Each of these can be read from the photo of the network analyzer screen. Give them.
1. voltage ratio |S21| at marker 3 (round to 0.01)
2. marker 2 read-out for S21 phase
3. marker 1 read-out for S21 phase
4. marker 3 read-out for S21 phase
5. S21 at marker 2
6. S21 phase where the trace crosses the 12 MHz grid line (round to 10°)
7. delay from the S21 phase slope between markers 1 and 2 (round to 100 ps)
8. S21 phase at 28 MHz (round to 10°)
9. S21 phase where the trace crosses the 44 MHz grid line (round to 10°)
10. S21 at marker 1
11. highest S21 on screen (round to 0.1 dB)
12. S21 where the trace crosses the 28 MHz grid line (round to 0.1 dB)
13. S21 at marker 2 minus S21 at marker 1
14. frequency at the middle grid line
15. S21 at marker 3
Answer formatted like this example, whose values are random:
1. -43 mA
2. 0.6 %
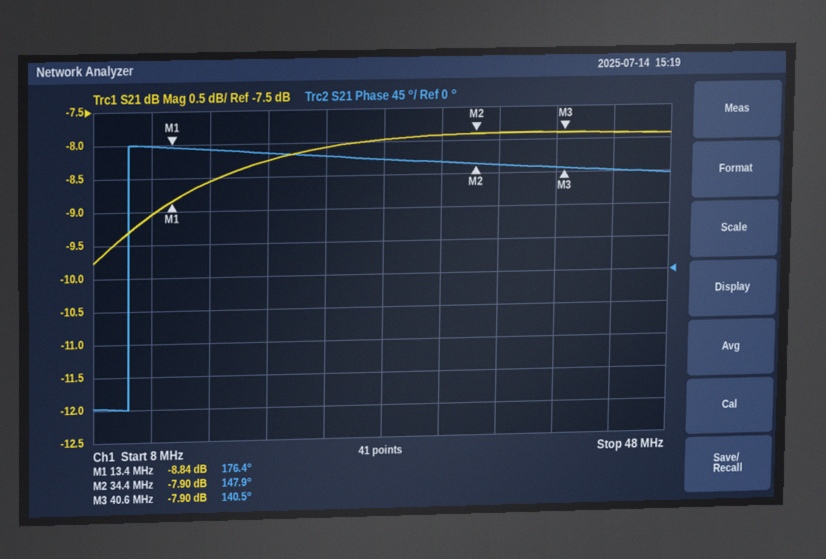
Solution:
1. 0.40
2. 147.9°
3. 176.4°
4. 140.5°
5. -7.90 dB
6. 180°
7. 3.8 ns
8. 160°
9. 140°
10. -8.84 dB
11. -7.9 dB
12. -8.0 dB
13. 0.94 dB
14. 28 MHz
15. -7.90 dB
